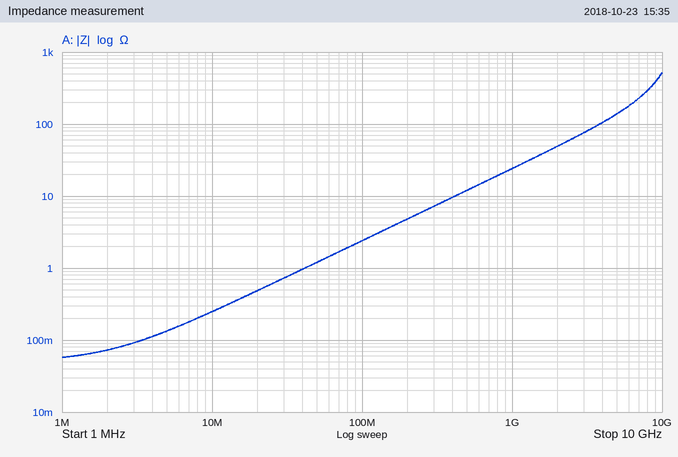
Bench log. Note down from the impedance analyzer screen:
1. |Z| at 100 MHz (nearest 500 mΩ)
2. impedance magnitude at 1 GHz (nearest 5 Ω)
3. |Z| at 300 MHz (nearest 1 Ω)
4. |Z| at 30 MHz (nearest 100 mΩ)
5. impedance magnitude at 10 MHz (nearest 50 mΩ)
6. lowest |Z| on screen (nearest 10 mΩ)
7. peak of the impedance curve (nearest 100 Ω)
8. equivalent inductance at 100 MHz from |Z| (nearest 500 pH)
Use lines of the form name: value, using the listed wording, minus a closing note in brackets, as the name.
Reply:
|Z| at 100 MHz: 2.5 Ω
impedance magnitude at 1 GHz: 25 Ω
|Z| at 300 MHz: 7 Ω
|Z| at 30 MHz: 700 mΩ
impedance magnitude at 10 MHz: 250 mΩ
lowest |Z| on screen: 60 mΩ
peak of the impedance curve: 500 Ω
equivalent inductance at 100 MHz from |Z|: 4.0 nH
